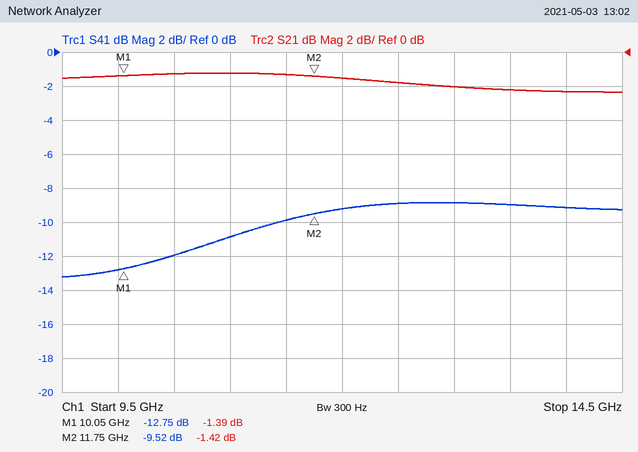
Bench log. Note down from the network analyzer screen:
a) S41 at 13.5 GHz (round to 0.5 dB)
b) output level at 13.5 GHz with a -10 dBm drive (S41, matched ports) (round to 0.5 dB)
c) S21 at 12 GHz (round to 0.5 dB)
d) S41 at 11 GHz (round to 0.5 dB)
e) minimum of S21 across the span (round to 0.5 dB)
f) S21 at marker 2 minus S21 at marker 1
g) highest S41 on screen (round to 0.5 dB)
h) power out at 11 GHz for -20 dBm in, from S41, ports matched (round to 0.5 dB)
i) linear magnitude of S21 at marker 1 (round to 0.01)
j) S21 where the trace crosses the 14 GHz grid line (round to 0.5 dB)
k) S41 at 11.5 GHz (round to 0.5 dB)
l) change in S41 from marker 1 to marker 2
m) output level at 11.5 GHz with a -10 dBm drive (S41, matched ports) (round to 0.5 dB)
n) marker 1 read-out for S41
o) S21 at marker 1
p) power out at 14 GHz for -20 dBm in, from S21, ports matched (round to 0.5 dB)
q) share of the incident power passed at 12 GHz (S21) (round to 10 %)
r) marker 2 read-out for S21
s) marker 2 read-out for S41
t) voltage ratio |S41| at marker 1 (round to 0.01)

-9.0 dB
-19.0 dBm
-1.5 dB
-11.0 dB
-2.5 dB
-0.03 dB
-9.0 dB
-31.0 dBm
0.85
-2.5 dB
-10.0 dB
3.23 dB
-20.0 dBm
-12.75 dB
-1.39 dB
-22.5 dBm
70 %
-1.42 dB
-9.52 dB
0.23
